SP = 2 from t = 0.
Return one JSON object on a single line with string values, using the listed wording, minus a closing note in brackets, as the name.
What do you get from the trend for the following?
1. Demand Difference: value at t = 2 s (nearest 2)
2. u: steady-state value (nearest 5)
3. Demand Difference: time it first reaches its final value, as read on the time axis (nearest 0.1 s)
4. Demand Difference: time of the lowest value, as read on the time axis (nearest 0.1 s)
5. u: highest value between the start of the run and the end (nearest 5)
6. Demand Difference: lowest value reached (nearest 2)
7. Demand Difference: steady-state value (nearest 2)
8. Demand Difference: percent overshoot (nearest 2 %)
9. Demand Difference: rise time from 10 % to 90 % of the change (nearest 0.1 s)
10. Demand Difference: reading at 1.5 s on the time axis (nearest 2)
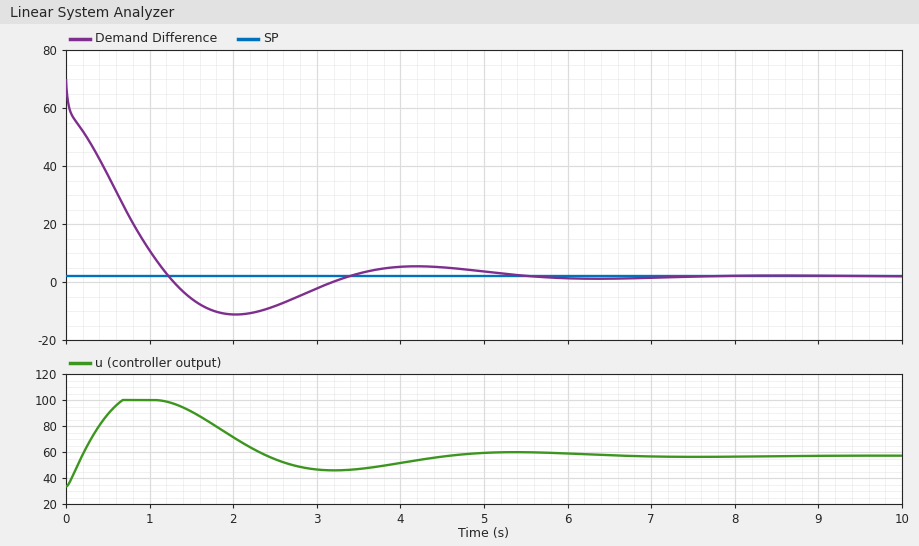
{"Demand Difference: value at t = 2 s": "-12", "u: steady-state value": "55", "Demand Difference: time it first reaches its final value, as read on the time axis": "1.2 s", "Demand Difference: time of the lowest value, as read on the time axis": "2.0 s", "u: highest value between the start of the run and the end": "100", "Demand Difference: lowest value reached": "-12", "Demand Difference: steady-state value": "2", "Demand Difference: percent overshoot": "20 %", "Demand Difference: rise time from 10 % to 90 % of the change": "1.0 s", "Demand Difference: reading at 1.5 s on the time axis": "-6"}
